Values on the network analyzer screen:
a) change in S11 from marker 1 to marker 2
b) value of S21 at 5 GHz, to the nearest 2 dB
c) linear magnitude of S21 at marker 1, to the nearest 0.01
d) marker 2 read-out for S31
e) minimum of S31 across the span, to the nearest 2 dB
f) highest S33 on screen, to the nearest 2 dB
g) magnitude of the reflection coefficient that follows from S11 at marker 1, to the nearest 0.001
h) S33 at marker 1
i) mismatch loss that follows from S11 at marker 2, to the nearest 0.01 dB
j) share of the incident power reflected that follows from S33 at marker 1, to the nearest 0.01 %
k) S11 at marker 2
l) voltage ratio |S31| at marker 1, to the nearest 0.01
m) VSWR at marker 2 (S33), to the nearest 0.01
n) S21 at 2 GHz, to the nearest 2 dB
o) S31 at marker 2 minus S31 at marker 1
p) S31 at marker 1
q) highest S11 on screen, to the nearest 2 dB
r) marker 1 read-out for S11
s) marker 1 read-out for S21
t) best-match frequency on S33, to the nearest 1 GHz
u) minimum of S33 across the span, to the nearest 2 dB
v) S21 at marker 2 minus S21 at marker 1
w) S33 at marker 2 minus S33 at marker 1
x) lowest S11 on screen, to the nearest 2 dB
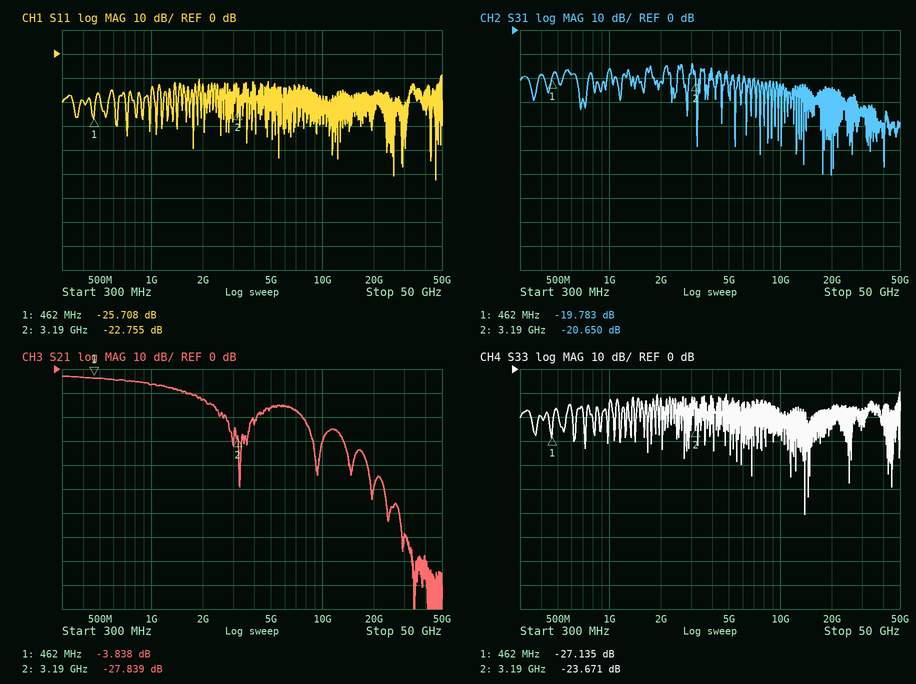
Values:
2.953 dB
-16 dB
0.64
-20.650 dB
-60 dB
-10 dB
0.052
-27.135 dB
0.02 dB
0.19 %
-22.755 dB
0.10
1.14
-12 dB
-0.867 dB
-19.783 dB
-8 dB
-25.708 dB
-3.838 dB
14 GHz
-60 dB
-24.001 dB
3.464 dB
-52 dB
